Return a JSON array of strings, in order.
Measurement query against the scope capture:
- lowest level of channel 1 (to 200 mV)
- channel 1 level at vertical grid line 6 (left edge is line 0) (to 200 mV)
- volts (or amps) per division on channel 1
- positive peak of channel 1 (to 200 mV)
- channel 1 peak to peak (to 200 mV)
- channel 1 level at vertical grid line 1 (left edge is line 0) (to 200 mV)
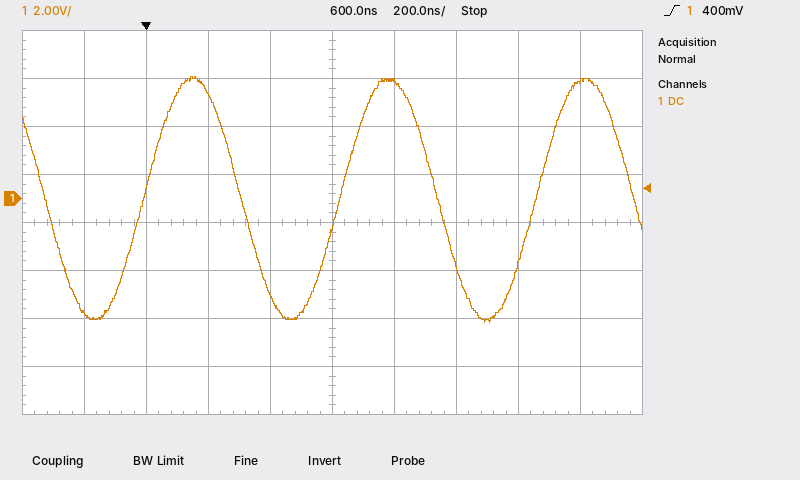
["-5.2 V", "4.8 V", "2 V", "5.0 V", "10.2 V", "-4.8 V"]
